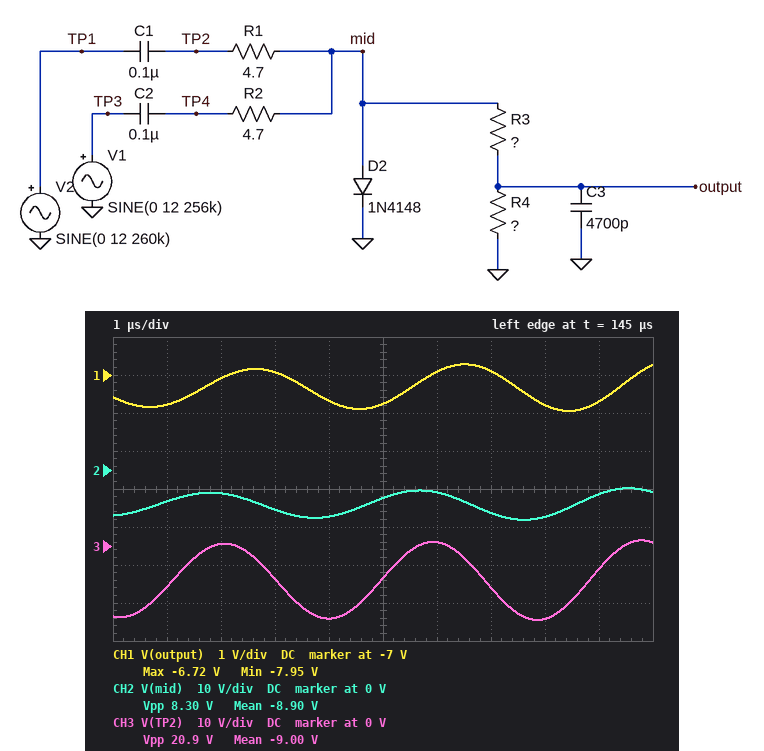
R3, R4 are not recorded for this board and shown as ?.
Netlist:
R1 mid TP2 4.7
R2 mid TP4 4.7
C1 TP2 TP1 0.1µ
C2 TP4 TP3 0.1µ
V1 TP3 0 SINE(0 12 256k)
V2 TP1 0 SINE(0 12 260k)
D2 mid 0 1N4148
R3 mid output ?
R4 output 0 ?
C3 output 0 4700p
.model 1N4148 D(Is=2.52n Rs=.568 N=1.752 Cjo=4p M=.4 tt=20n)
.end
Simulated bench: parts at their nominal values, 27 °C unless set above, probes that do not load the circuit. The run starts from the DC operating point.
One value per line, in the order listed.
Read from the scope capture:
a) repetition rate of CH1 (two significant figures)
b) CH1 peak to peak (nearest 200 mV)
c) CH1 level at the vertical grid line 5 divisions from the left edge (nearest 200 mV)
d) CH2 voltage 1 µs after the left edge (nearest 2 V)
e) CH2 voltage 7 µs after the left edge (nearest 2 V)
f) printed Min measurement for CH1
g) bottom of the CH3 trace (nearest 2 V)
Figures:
260 kHz
1.2 V
-7.8 V
-8 V
-12 V
-7.95 V
-20 V
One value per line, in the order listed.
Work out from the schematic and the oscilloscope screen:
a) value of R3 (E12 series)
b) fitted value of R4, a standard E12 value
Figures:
820 Ω
3.3 kΩ
